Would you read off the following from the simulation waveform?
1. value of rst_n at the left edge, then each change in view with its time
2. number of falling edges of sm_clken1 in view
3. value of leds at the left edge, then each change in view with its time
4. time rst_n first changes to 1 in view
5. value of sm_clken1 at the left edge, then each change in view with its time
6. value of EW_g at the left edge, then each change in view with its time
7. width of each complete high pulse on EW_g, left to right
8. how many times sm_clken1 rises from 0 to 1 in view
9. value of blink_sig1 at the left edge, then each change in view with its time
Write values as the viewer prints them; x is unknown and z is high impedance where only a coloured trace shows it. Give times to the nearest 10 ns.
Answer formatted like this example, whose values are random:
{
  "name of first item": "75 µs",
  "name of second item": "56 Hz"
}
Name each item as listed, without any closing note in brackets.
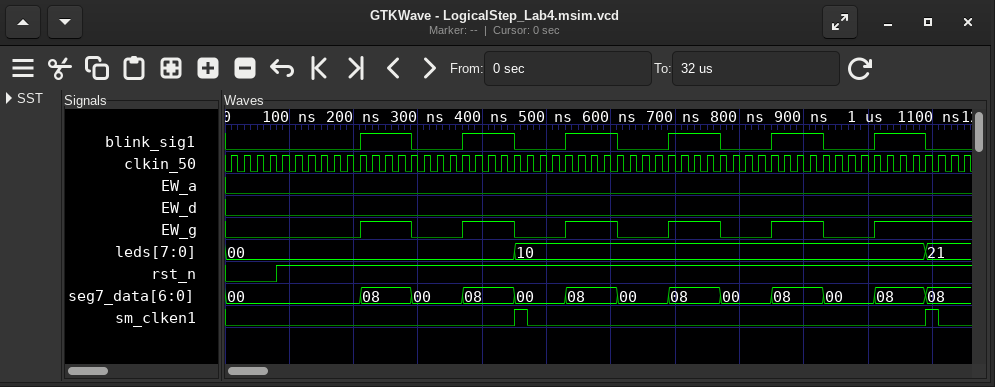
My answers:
{
  "value of rst_n at the left edge, then each change in view with its time": "0, 1 at 80 ns",
  "number of falling edges of sm_clken1 in view": "2",
  "value of leds at the left edge, then each change in view with its time": "00, 10 at 450 ns, 21 at 1090 ns",
  "time rst_n first changes to 1 in view": "80 ns",
  "value of sm_clken1 at the left edge, then each change in view with its time": "0, 1 at 450 ns, 0 at 470 ns, 1 at 1090 ns, 0 at 1110 ns",
  "value of EW_g at the left edge, then each change in view with its time": "0, 1 at 210 ns, 0 at 290 ns, 1 at 370 ns, 0 at 450 ns, 1 at 530 ns, 0 at 610 ns, 1 at 690 ns, 0 at 770 ns, 1 at 850 ns, 0 at 930 ns, 1 at 1010 ns",
  "width of each complete high pulse on EW_g, left to right": "80 ns, 80 ns, 80 ns, 80 ns, 80 ns",
  "how many times sm_clken1 rises from 0 to 1 in view": "2",
  "value of blink_sig1 at the left edge, then each change in view with its time": "0, 1 at 210 ns, 0 at 290 ns, 1 at 370 ns, 0 at 450 ns, 1 at 530 ns, 0 at 610 ns, 1 at 690 ns, 0 at 770 ns, 1 at 850 ns, 0 at 930 ns, 1 at 1010 ns, 0 at 1090 ns"
}
